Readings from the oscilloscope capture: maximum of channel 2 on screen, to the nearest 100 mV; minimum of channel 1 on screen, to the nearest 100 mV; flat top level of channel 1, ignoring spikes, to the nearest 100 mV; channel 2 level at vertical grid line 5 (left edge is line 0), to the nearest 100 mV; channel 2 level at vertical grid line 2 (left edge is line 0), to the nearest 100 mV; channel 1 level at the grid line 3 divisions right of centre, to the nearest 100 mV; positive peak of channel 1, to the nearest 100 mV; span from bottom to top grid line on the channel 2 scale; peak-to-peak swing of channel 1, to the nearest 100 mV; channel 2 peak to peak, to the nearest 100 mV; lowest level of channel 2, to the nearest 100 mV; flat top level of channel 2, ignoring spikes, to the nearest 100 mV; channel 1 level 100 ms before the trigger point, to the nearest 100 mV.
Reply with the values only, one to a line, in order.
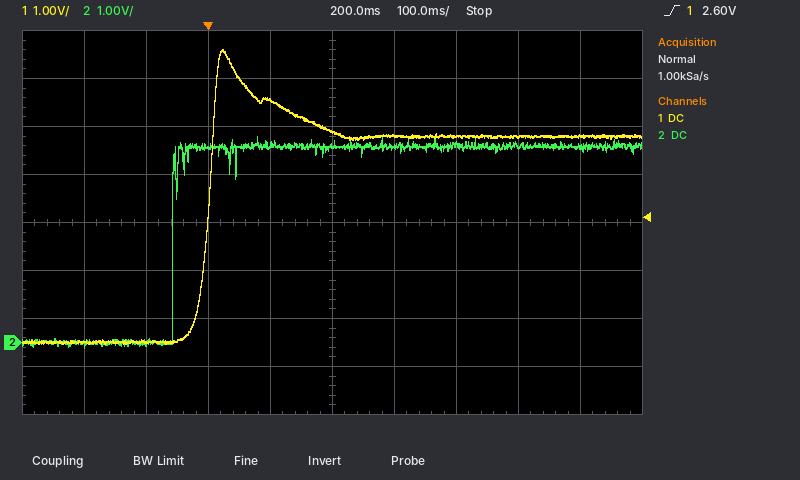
4.3 V
0.0 V
4.3 V
4.1 V
0.0 V
4.3 V
6.1 V
8 V
6.1 V
4.4 V
-100 mV
4.1 V
0.0 V
